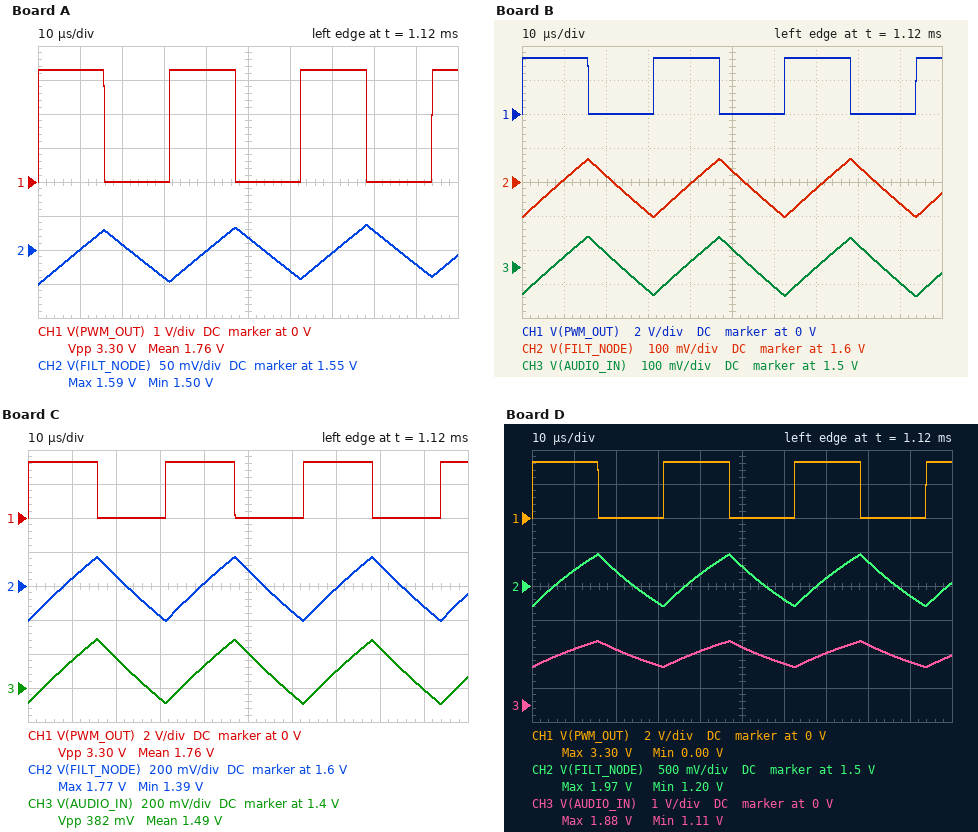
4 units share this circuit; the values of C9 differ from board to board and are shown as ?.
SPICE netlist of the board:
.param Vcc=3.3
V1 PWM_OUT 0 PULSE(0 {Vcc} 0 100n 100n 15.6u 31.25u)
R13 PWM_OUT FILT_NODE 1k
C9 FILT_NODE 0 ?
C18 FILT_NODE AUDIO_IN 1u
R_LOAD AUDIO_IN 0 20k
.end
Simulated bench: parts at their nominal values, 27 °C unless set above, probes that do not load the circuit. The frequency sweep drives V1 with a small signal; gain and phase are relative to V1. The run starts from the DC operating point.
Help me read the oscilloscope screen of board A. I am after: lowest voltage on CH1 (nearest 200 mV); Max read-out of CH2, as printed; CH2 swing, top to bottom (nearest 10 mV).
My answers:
0 V
1.59 V
90 mV
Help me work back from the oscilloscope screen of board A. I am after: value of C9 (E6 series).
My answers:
330 nF
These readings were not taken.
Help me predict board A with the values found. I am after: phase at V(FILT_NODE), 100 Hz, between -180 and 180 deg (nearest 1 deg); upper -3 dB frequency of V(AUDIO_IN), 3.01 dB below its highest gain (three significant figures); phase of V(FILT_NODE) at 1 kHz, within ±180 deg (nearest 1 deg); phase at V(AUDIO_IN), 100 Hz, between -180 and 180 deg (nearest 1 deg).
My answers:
-11 deg
522 Hz
-63 deg
-7 deg
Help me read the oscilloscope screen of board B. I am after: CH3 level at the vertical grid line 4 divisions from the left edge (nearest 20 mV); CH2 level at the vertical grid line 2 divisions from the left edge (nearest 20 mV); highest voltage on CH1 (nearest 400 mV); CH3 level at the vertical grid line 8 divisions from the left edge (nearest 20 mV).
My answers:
1.52 V
1.62 V
3.2 V
1.56 V
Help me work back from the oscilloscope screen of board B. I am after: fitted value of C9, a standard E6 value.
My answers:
150 nF
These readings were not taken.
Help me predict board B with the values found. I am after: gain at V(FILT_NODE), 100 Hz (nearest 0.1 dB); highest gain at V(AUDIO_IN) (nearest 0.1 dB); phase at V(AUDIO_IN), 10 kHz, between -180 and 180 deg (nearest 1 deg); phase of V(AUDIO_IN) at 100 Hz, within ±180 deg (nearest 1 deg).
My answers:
-0.5 dB
-0.5 dB
-84 deg
-1 deg
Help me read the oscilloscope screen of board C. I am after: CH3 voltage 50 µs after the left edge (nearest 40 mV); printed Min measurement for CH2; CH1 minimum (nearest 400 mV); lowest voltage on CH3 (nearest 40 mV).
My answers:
1.60 V
1.39 V
0 V
1.32 V
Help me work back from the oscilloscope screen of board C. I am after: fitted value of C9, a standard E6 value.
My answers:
68 nF
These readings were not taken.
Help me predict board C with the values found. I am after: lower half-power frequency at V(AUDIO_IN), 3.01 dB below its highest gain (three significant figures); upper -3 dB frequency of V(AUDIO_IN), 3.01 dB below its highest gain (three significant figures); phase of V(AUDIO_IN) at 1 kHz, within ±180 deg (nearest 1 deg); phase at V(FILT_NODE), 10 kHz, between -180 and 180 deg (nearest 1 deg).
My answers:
7.53 Hz
2.47 kHz
-22 deg
-76 deg
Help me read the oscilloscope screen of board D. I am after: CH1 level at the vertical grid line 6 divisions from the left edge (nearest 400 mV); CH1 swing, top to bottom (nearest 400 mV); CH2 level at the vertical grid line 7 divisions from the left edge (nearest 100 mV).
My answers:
0 V
3.2 V
1.6 V
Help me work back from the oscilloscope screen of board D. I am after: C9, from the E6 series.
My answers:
33 nF
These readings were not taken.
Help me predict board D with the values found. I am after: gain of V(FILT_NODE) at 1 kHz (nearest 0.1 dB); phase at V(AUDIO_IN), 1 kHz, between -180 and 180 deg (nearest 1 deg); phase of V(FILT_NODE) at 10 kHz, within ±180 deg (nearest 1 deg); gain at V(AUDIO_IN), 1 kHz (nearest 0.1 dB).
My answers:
-0.6 dB
-11 deg
-63 deg
-0.6 dB
